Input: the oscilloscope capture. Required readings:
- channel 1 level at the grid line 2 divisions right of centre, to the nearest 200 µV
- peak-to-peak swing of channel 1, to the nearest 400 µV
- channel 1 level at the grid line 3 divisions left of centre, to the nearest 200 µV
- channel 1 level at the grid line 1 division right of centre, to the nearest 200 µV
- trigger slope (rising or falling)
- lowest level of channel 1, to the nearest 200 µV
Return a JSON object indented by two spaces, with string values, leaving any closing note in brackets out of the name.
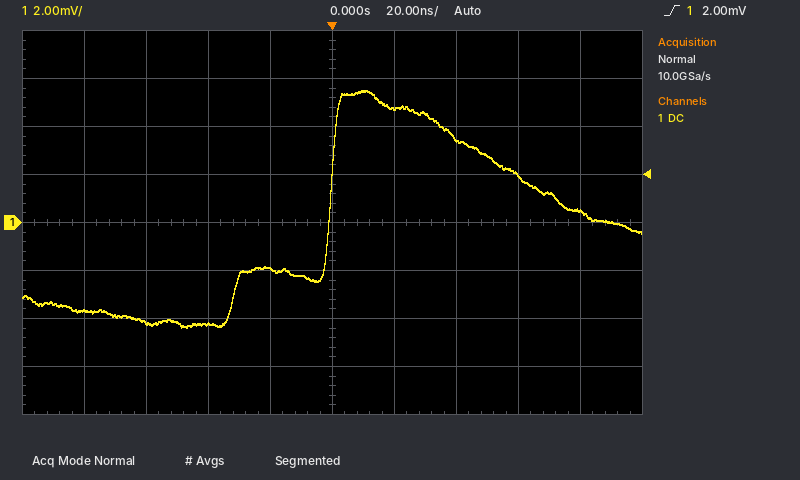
{
  "channel 1 level at the grid line 2 divisions right of centre, to the nearest 200 µV": "3.4 mV",
  "peak-to-peak swing of channel 1, to the nearest 400 µV": "10.0 mV",
  "channel 1 level at the grid line 3 divisions left of centre, to the nearest 200 µV": "-4.2 mV",
  "channel 1 level at the grid line 1 division right of centre, to the nearest 200 µV": "4.8 mV",
  "trigger slope": "rising",
  "lowest level of channel 1, to the nearest 200 µV": "-4.4 mV"
}
